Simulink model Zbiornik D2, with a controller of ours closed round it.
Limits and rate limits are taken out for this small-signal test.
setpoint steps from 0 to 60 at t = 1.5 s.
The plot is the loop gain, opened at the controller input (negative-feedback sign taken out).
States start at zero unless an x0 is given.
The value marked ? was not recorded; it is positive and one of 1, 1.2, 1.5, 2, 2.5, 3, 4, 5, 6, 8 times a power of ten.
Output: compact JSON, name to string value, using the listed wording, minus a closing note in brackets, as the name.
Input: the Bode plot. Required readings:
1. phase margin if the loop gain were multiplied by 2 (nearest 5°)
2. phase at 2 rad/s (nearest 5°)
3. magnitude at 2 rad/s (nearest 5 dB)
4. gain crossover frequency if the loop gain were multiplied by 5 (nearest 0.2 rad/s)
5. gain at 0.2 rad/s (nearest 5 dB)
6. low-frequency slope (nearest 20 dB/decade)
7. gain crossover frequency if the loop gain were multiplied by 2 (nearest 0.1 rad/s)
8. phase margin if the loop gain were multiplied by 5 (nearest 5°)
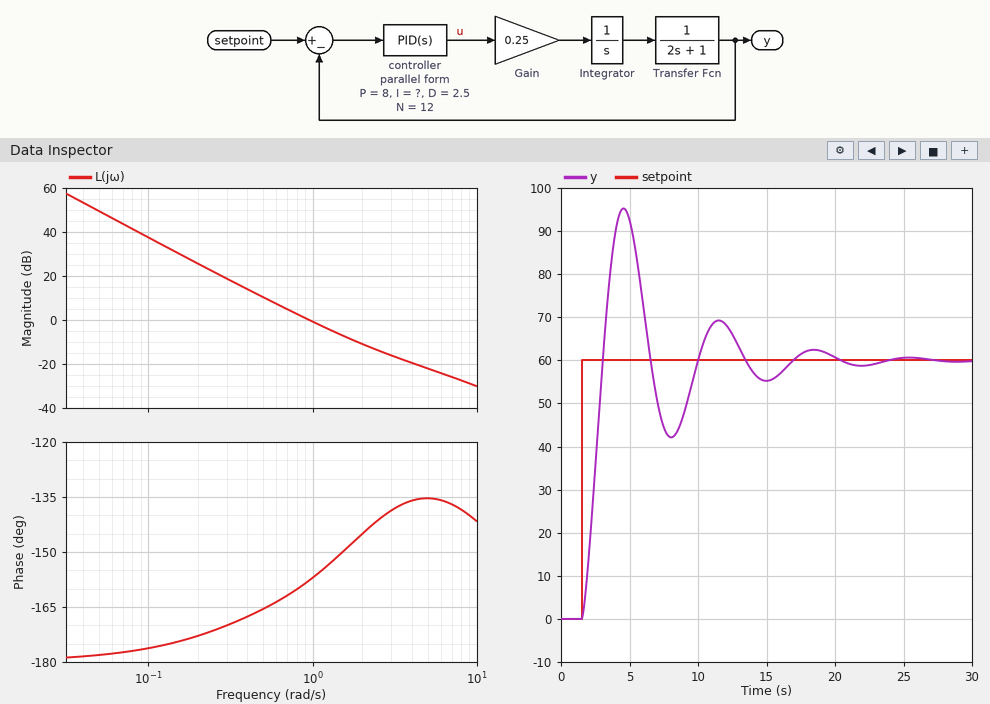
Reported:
{"phase margin if the loop gain were multiplied by 2": "30°", "phase at 2 rad/s": "-145°", "magnitude at 2 rad/s": "-10 dB", "gain crossover frequency if the loop gain were multiplied by 5": "2.6 rad/s", "gain at 0.2 rad/s": "25 dB", "low-frequency slope": "-40 dB/decade", "gain crossover frequency if the loop gain were multiplied by 2": "1.4 rad/s", "phase margin if the loop gain were multiplied by 5": "40°"}
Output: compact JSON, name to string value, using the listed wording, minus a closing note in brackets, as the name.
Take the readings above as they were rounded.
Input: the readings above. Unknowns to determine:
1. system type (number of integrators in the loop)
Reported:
{"system type": "2"}
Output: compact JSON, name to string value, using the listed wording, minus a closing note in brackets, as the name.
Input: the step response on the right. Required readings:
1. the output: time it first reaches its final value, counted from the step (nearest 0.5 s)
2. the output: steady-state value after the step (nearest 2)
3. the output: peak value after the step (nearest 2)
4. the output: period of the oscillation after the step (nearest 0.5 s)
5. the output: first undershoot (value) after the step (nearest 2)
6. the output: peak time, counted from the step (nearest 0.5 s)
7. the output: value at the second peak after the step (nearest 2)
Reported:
{"the output: time it first reaches its final value, counted from the step": "1.5 s", "the output: steady-state value after the step": "60", "the output: peak value after the step": "96", "the output: period of the oscillation after the step": "7.0 s", "the output: first undershoot (value) after the step": "42", "the output: peak time, counted from the step": "3.0 s", "the output: value at the second peak after the step": "70"}
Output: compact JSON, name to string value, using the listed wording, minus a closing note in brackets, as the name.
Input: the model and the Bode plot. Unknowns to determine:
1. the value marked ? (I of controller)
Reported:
{"the value marked ?": "3"}
